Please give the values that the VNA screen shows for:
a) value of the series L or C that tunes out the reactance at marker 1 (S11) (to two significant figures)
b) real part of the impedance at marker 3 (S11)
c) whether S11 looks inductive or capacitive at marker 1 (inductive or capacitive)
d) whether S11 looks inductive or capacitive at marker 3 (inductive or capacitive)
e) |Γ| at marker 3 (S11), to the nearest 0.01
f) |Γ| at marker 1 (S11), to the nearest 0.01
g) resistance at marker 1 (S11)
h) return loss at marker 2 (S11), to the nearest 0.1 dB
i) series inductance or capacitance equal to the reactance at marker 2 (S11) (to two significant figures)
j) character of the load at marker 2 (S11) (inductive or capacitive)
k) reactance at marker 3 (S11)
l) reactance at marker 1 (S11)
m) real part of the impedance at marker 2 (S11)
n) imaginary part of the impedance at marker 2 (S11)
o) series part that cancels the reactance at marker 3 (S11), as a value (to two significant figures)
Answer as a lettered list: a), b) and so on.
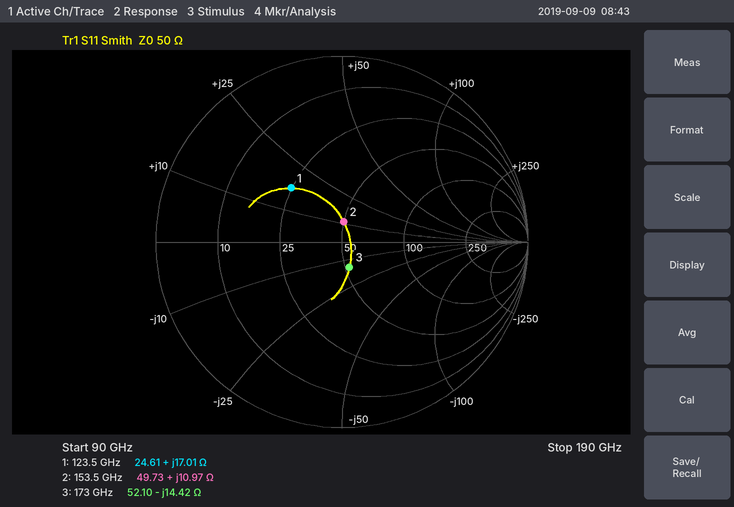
a) 76 fF
b) 52.10 Ω
c) inductive
d) capacitive
e) 0.14
f) 0.40
g) 24.61 Ω
h) 19.2 dB
i) 11 pH
j) inductive
k) -14.42 Ω
l) +17.01 Ω
m) 49.73 Ω
n) +10.97 Ω
o) 13 pH
